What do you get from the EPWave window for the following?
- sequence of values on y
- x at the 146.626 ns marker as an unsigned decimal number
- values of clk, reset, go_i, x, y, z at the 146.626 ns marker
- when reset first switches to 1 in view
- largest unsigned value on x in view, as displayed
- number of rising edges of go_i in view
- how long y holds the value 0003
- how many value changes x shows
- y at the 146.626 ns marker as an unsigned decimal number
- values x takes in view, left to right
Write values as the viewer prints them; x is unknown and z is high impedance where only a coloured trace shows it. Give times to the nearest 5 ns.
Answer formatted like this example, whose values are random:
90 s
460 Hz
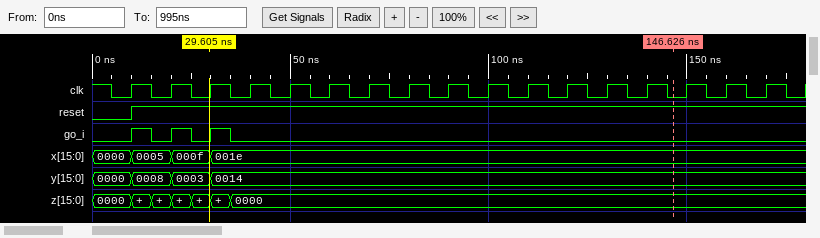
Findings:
0000, 0008, 0003, 0014
30
clk=0, reset=1, go_i=0, x=001e, y=0014, z=0000
10 ns
001e
3
10 ns
3
20
0000, 0005, 000f, 001e
